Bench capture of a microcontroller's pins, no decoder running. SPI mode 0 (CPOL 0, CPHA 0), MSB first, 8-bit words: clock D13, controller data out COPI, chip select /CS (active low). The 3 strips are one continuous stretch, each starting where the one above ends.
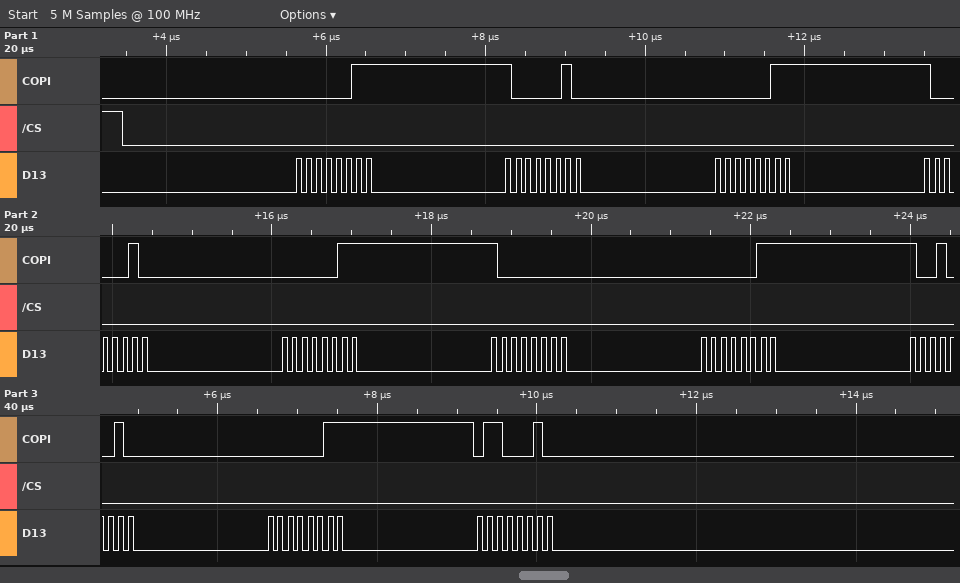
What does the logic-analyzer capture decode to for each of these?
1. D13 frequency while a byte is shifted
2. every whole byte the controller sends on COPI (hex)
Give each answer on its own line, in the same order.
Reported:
8 MHz
0x03 0x82 0x03 0x82 0x03 0x80 0x03 0x92 0x03 0x62
